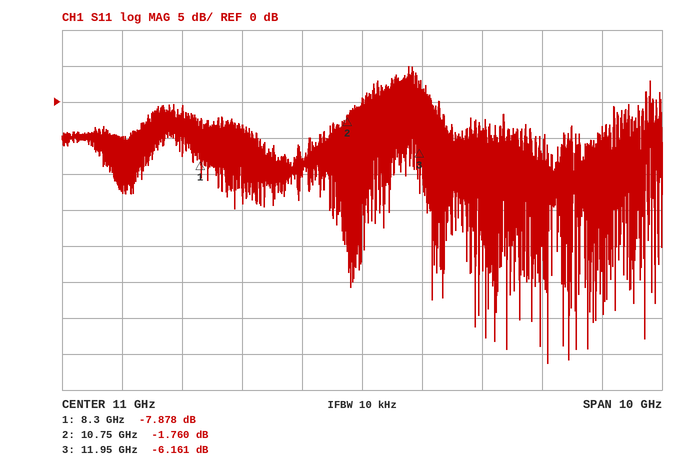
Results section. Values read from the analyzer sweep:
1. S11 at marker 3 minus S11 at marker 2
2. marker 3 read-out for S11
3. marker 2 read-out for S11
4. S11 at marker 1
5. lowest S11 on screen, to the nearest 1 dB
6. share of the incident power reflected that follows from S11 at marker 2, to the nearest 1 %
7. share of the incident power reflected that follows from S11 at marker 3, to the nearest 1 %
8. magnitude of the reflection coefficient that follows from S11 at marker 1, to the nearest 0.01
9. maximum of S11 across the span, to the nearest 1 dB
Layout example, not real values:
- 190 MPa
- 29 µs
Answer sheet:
- -4.401 dB
- -6.161 dB
- -1.760 dB
- -7.878 dB
- -36 dB
- 67 %
- 24 %
- 0.40
- 5 dB
